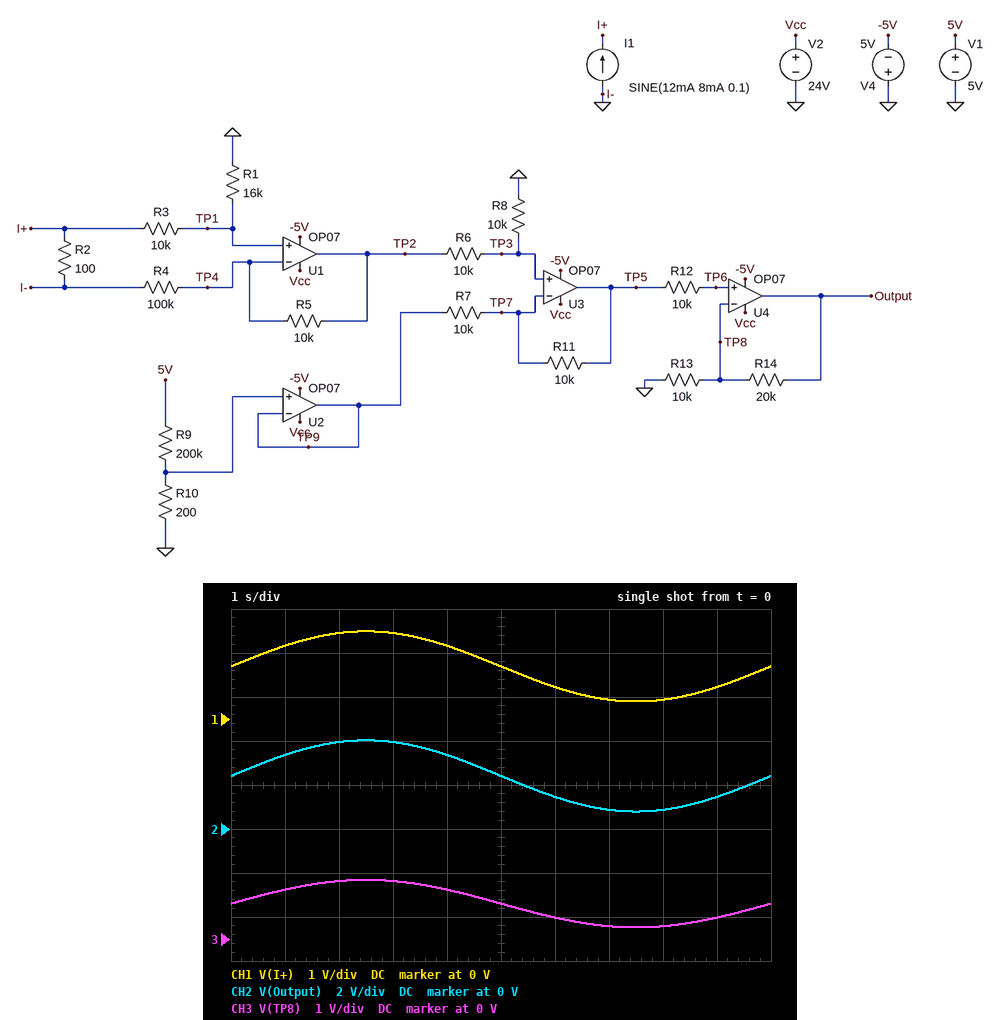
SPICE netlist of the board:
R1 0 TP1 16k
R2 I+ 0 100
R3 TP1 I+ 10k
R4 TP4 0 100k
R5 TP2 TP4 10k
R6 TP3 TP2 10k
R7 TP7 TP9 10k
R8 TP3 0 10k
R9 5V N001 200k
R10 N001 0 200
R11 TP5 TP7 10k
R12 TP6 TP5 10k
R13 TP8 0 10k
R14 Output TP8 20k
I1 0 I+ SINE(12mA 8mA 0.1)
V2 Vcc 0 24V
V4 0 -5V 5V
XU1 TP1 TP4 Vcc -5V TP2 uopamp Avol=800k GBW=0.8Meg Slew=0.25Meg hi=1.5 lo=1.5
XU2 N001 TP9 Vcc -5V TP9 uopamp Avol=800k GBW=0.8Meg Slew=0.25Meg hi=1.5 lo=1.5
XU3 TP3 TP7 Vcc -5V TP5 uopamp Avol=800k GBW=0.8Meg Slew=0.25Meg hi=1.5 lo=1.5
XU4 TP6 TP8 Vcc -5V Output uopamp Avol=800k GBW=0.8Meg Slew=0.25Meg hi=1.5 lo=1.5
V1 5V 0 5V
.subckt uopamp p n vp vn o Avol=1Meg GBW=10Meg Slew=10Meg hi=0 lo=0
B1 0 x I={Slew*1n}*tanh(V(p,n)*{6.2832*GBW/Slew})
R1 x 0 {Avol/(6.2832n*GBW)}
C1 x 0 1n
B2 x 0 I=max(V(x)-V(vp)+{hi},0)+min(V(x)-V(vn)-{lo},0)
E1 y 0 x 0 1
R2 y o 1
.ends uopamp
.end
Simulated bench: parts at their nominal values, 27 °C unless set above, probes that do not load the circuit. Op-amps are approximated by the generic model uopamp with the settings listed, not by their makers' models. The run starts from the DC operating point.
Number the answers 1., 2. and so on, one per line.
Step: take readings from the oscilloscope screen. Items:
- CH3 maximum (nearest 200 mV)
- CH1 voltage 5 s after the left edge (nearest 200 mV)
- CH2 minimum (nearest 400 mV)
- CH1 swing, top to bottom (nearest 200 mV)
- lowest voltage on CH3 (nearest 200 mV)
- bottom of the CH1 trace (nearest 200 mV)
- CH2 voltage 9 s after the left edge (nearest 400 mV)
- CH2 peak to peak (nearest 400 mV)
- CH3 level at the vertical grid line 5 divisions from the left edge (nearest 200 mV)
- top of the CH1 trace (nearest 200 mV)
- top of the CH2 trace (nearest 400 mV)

1. 1.4 V
2. 1.2 V
3. 800 mV
4. 1.6 V
5. 200 mV
6. 400 mV
7. 1.6 V
8. 3.2 V
9. 800 mV
10. 2.0 V
11. 4.0 V
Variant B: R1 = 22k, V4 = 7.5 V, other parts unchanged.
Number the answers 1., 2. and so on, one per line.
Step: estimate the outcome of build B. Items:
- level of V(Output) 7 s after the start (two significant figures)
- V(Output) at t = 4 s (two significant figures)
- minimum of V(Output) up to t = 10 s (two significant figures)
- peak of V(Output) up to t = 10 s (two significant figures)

1. 980 mV
2. 3.8 V
3. 890 mV
4. 4.5 V
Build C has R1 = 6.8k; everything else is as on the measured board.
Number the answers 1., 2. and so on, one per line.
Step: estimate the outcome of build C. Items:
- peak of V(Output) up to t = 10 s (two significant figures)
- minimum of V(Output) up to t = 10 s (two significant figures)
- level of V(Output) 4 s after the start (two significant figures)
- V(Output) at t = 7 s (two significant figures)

1. 2.6 V
2. 520 mV
3. 2.2 V
4. 570 mV
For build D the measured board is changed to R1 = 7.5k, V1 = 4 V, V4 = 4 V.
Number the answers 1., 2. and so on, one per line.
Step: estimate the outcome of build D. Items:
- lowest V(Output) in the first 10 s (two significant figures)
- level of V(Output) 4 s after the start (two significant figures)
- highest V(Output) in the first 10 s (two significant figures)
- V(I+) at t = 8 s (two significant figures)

1. 550 mV
2. 2.3 V
3. 2.8 V
4. 440 mV
